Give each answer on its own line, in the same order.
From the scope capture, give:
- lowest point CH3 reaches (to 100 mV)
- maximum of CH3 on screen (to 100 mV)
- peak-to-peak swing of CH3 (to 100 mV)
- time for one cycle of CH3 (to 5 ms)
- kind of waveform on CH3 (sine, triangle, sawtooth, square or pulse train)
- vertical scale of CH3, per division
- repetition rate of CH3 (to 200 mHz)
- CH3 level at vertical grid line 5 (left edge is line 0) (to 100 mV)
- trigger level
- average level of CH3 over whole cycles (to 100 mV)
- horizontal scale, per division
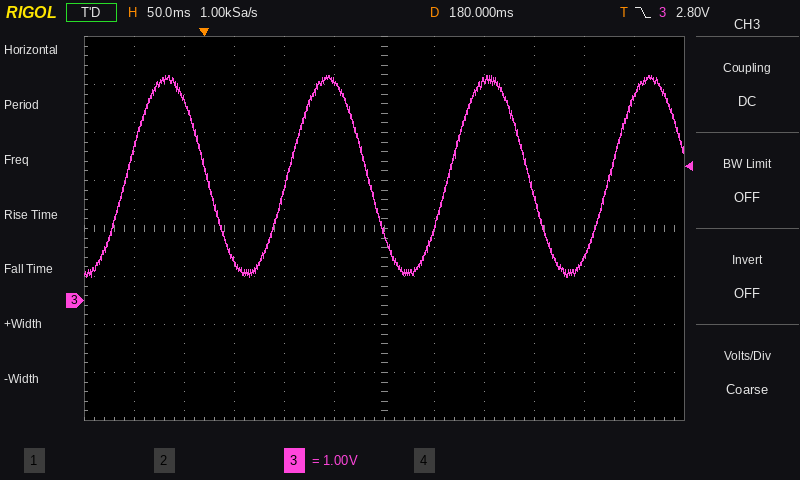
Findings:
500 mV
4.7 V
4.2 V
160 ms
sine
1 V
6.2 Hz
4.6 V
2.80 V
2.6 V
50 ms
